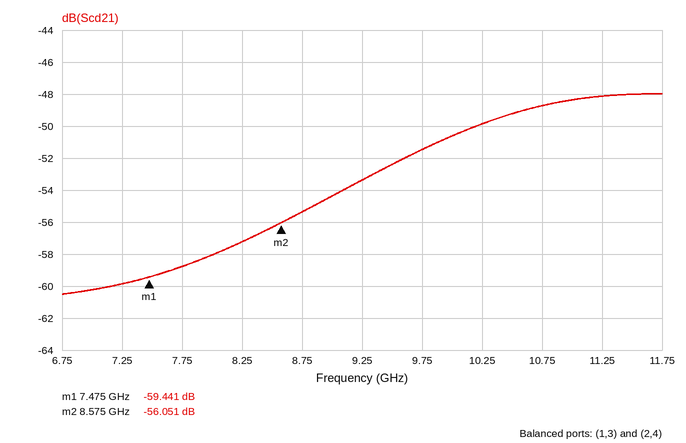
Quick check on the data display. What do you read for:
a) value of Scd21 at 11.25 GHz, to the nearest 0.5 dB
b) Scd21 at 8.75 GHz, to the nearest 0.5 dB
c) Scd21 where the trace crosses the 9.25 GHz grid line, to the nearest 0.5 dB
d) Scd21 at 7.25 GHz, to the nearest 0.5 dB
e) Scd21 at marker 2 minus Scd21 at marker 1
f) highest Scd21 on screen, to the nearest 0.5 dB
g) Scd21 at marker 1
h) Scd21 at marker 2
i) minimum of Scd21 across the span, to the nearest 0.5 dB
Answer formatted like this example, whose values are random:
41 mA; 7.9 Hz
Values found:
-48.0 dB; -55.5 dB; -53.5 dB; -60.0 dB; 3.390 dB; -48.0 dB; -59.441 dB; -56.051 dB; -60.5 dB
